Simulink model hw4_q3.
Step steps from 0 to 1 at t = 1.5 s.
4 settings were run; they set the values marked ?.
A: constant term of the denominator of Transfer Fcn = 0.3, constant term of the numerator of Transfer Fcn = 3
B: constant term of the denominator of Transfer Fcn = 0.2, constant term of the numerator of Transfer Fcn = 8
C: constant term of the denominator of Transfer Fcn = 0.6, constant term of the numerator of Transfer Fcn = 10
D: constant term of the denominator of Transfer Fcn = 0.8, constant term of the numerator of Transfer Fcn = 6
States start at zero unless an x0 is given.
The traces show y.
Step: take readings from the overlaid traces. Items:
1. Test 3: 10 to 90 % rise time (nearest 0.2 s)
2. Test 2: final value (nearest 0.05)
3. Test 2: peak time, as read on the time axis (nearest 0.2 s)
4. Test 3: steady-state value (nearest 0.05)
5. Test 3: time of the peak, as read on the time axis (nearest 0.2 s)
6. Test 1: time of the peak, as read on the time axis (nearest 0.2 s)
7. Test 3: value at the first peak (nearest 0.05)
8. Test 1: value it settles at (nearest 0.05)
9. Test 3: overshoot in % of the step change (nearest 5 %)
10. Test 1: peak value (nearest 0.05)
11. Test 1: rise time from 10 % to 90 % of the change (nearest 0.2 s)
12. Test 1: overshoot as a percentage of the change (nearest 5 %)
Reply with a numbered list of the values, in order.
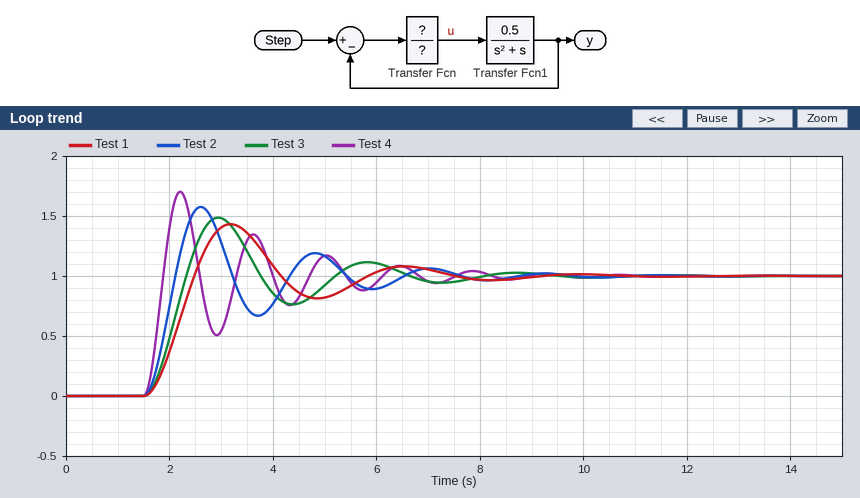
1. 0.6 s
2. 1.00
3. 2.6 s
4. 1.00
5. 3.0 s
6. 3.2 s
7. 1.50
8. 1.00
9. 50 %
10. 1.45
11. 0.6 s
12. 45 %
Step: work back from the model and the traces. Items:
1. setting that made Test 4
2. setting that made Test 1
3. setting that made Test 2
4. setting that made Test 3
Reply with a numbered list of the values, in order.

1. B
2. D
3. C
4. A
